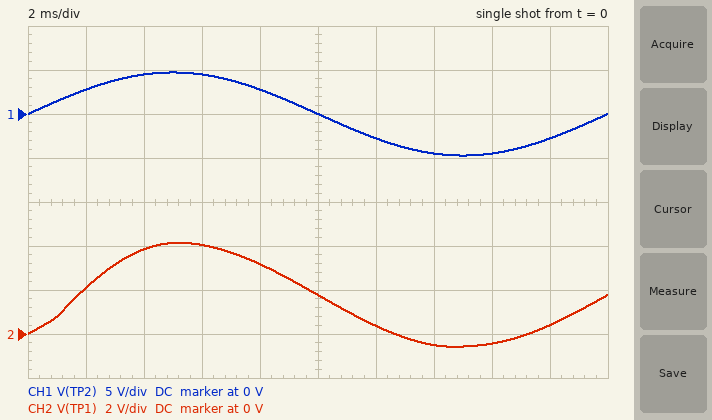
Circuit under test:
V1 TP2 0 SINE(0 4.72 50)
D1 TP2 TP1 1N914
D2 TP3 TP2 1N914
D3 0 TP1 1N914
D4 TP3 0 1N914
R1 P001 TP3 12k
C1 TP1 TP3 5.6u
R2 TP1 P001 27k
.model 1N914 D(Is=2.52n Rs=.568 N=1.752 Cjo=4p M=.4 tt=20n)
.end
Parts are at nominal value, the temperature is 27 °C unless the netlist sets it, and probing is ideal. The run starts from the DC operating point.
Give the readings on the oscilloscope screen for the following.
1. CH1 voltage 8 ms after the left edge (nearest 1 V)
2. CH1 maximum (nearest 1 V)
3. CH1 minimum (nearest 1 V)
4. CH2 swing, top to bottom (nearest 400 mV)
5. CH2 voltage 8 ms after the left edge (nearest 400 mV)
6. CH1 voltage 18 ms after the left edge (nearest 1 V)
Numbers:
3 V
5 V
-5 V
4.8 V
3.2 V
-3 V
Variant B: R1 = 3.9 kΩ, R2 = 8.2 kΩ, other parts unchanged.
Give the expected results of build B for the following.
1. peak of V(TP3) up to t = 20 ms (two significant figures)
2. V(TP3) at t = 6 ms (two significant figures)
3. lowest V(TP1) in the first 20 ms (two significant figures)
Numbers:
680 mV
460 mV
-620 mV
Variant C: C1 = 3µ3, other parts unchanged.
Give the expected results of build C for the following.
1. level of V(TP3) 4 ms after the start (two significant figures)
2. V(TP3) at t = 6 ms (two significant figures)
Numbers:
610 mV
420 mV
